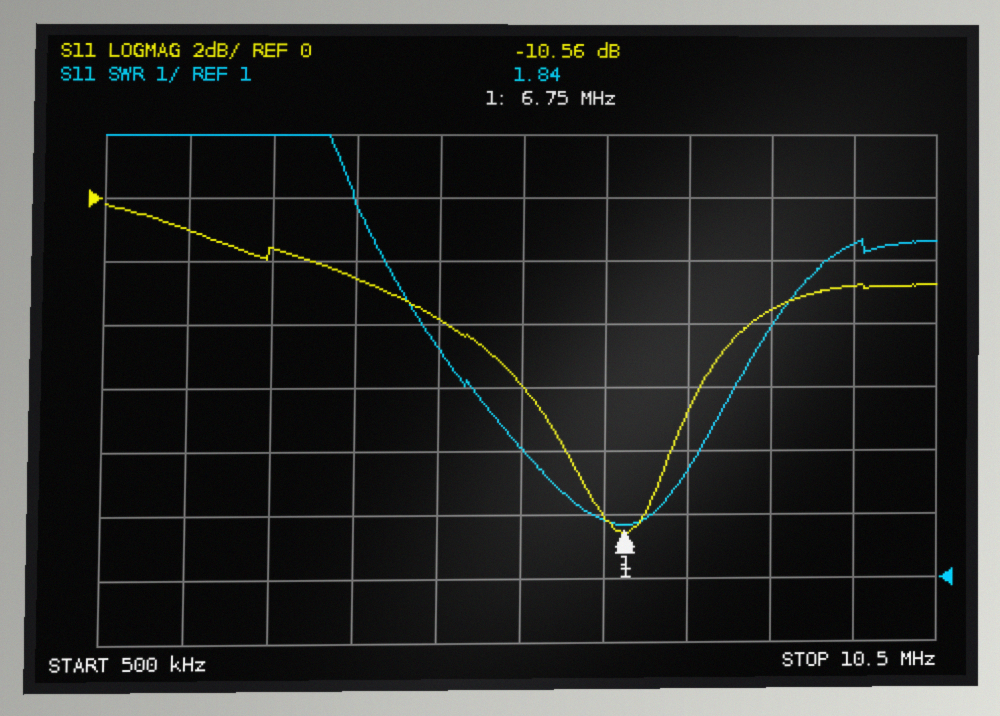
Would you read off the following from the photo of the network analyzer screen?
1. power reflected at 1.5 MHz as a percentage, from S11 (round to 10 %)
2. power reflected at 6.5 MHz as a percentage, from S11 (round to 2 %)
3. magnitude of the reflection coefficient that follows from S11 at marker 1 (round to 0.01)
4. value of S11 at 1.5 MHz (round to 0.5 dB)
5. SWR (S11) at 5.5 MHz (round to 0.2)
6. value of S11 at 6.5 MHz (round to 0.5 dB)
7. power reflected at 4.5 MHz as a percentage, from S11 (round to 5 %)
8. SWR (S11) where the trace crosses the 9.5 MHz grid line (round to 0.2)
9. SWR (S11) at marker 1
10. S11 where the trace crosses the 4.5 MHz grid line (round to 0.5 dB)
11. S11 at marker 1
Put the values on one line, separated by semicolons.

80 %; 10 %; 0.30; -1.0 dB; 3.0; -10.0 dB; 40 %; 6.2; 1.84; -4.0 dB; -10.56 dB
